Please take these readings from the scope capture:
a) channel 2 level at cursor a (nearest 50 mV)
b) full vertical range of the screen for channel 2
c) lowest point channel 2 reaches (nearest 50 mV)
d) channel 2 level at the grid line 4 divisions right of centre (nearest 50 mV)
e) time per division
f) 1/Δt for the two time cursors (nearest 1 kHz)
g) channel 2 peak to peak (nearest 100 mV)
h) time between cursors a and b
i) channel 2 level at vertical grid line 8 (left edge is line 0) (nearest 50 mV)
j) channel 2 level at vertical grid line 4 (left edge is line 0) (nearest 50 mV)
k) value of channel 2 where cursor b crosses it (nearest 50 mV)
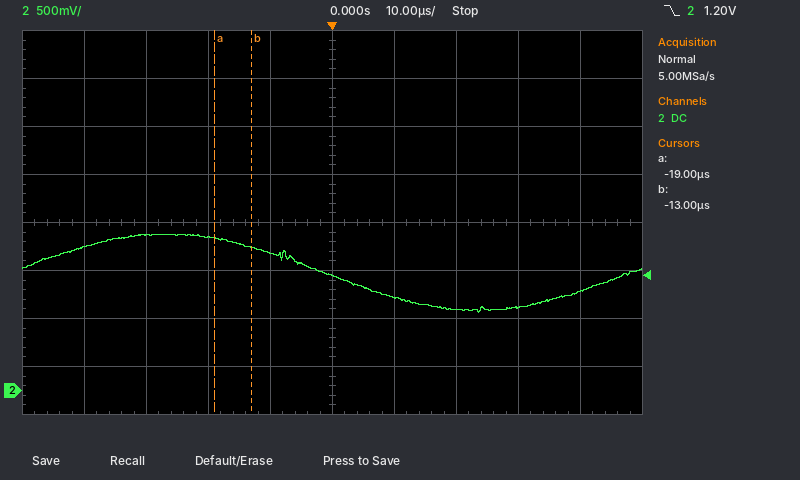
1.60 V
4 V
800 mV
1.05 V
10 µs
167 kHz
800 mV
6 µs
850 mV
1.45 V
1.50 V
